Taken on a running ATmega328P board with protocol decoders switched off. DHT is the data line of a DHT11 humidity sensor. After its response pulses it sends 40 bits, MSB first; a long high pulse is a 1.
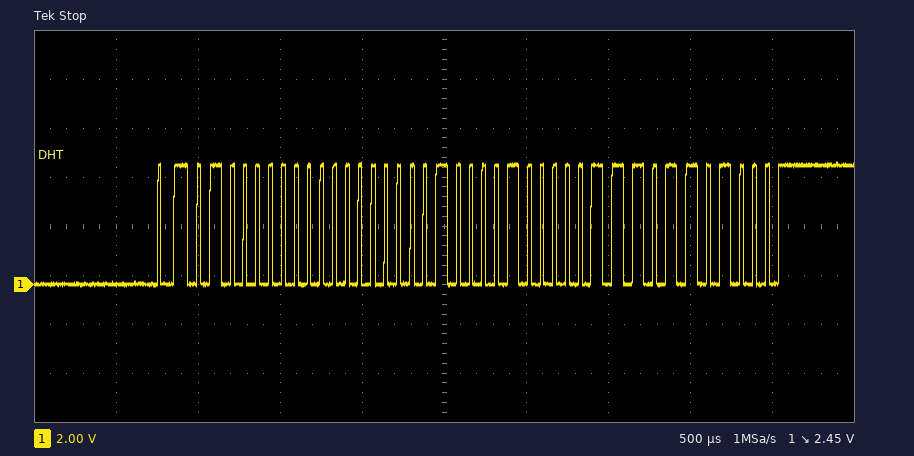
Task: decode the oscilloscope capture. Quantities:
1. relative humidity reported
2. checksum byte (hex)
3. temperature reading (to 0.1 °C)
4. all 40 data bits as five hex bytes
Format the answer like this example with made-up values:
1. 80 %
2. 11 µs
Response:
1. 64 %
2. 0x68
3. 33.7 °C
4. 40 00 21 07 68
